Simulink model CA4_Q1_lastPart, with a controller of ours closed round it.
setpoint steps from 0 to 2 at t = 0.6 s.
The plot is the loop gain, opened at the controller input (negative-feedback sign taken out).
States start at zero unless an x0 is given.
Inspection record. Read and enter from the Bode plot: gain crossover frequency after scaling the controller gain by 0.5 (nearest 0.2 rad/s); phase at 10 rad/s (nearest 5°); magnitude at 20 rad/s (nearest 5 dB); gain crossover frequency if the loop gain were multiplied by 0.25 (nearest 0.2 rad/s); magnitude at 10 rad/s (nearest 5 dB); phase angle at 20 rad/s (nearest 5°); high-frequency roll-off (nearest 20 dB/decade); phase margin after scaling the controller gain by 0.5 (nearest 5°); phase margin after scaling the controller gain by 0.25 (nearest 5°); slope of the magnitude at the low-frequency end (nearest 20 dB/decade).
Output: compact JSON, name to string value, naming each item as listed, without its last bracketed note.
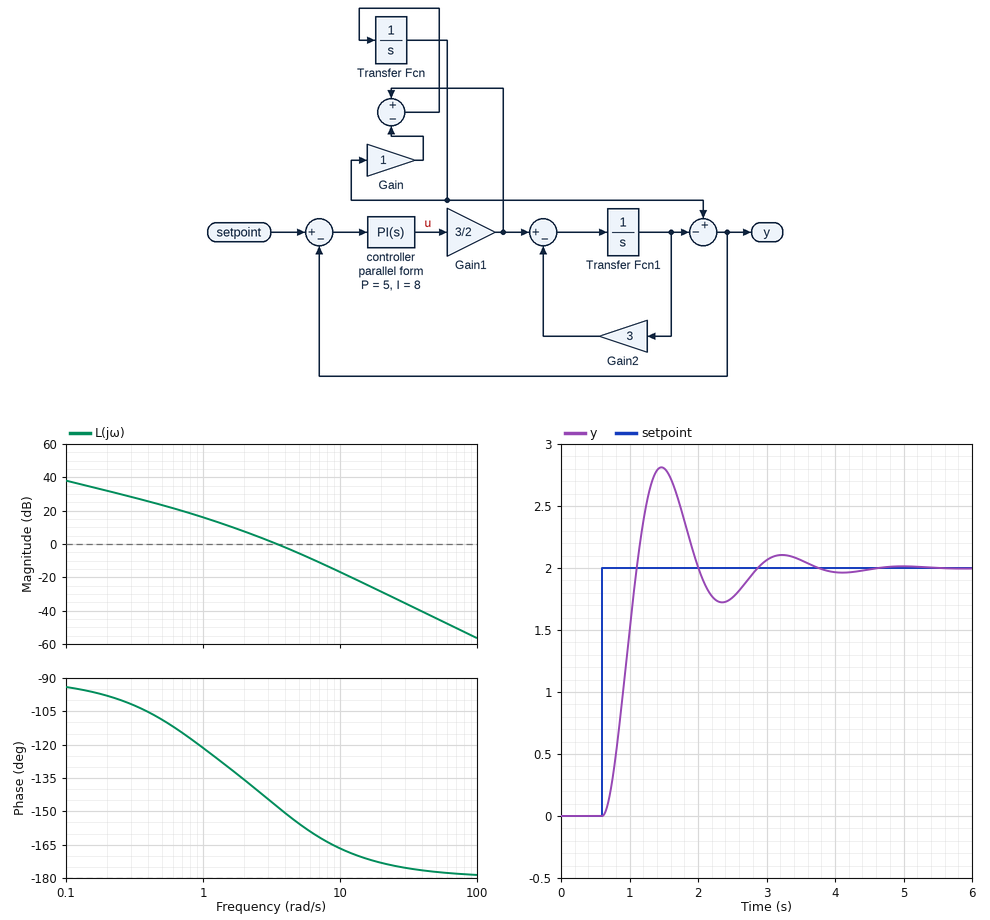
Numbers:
{"gain crossover frequency after scaling the controller gain by 0.5": "2.2 rad/s", "phase at 10 rad/s": "-165°", "magnitude at 20 rad/s": "-30 dB", "gain crossover frequency if the loop gain were multiplied by 0.25": "1.4 rad/s", "magnitude at 10 rad/s": "-15 dB", "phase angle at 20 rad/s": "-175°", "high-frequency roll-off": "-40 dB/decade", "phase margin after scaling the controller gain by 0.5": "40°", "phase margin after scaling the controller gain by 0.25": "50°", "slope of the magnitude at the low-frequency end": "-20 dB/decade"}
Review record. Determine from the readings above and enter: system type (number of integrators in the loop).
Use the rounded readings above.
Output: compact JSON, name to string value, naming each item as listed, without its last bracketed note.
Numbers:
{"system type": "1"}
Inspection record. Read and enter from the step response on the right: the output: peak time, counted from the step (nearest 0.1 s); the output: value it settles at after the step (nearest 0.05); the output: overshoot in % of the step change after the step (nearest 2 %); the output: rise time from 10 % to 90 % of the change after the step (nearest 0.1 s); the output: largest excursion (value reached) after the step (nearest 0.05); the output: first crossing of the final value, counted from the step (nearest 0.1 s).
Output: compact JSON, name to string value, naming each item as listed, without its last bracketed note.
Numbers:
{"the output: peak time, counted from the step": "0.9 s", "the output: value it settles at after the step": "2.00", "the output: overshoot in % of the step change after the step": "40 %", "the output: rise time from 10 % to 90 % of the change after the step": "0.3 s", "the output: largest excursion (value reached) after the step": "2.80", "the output: first crossing of the final value, counted from the step": "0.5 s"}
